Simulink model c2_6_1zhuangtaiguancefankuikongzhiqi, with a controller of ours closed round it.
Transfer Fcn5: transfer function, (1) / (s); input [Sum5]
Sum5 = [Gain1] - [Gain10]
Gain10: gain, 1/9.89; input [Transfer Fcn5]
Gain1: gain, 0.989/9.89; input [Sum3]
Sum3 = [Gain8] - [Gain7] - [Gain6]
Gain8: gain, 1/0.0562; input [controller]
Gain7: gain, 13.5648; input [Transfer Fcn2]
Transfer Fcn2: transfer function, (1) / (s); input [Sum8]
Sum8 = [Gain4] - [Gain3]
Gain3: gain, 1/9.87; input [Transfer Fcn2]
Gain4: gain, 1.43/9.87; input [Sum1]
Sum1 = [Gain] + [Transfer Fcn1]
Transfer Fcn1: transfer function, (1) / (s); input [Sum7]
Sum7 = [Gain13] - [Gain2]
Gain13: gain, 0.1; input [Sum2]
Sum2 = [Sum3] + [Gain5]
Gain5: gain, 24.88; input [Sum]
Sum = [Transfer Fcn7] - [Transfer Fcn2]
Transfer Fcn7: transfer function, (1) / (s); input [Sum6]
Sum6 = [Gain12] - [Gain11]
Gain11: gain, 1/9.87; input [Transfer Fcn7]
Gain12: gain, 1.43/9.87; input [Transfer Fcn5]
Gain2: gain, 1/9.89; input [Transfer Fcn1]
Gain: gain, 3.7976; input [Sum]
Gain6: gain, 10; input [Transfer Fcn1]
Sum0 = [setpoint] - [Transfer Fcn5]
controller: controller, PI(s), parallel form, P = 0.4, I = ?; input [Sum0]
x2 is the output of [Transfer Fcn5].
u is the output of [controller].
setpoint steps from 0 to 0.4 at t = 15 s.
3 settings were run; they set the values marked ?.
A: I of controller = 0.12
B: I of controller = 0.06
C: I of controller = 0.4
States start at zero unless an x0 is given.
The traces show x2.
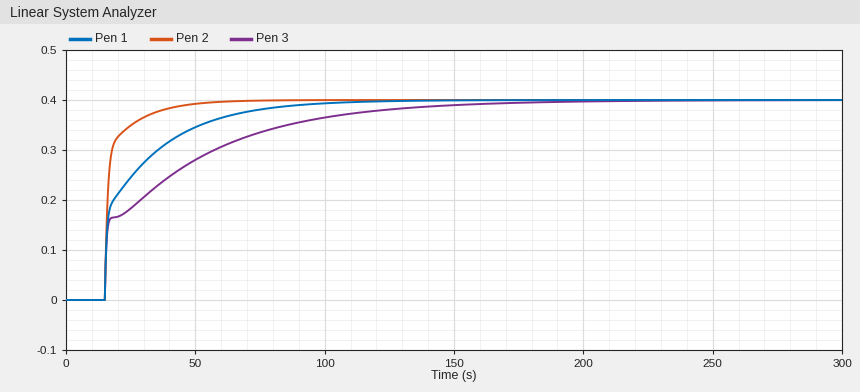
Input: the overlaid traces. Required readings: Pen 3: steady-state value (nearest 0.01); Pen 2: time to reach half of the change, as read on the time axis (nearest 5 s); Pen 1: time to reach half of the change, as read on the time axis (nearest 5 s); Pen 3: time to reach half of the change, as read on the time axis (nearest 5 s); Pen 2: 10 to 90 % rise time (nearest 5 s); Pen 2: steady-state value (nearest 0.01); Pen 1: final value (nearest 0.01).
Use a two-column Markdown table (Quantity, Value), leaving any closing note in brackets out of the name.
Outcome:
| Quantity | Value |
|---|---|
| Pen 3: steady-state value | 0.40 |
| Pen 2: time to reach half of the change, as read on the time axis | 15 s |
| Pen 1: time to reach half of the change, as read on the time axis | 20 s |
| Pen 3: time to reach half of the change, as read on the time axis | 30 s |
| Pen 2: 10 to 90 % rise time | 15 s |
| Pen 2: steady-state value | 0.40 |
| Pen 1: final value | 0.40 |
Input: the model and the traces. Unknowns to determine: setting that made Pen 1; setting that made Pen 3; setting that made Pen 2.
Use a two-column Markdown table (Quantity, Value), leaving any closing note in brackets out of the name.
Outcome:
| Quantity | Value |
|---|---|
| setting that made Pen 1 | A |
| setting that made Pen 3 | B |
| setting that made Pen 2 | C |
